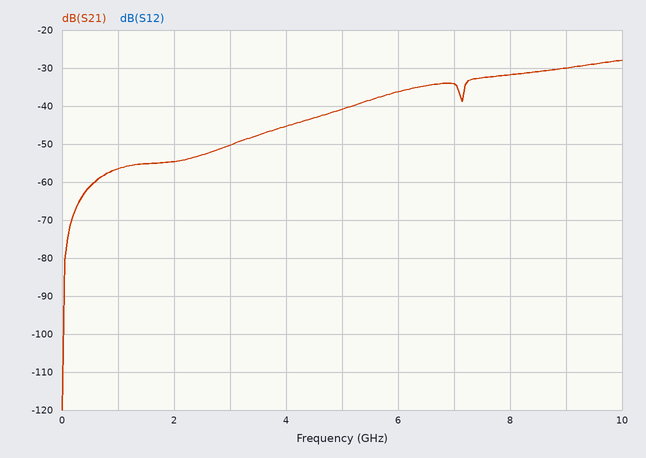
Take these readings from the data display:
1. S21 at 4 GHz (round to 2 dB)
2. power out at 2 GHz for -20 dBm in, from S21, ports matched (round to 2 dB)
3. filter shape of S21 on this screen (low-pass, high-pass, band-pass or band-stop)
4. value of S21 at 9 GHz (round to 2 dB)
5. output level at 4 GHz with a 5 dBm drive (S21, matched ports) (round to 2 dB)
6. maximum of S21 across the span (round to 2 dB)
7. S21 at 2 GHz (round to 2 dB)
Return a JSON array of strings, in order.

["-46 dB", "-74 dBm", "high-pass", "-30 dB", "-40 dBm", "-28 dB", "-54 dB"]
